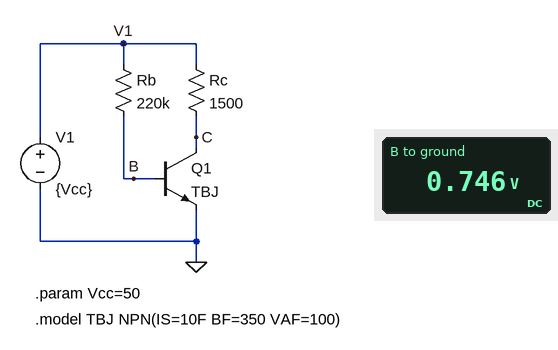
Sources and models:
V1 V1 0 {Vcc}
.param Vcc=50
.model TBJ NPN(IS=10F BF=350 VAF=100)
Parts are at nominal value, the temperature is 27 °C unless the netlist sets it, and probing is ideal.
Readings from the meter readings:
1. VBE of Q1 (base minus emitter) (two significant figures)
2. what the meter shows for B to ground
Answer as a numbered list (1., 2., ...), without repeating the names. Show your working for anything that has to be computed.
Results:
1. 746 mV = 750 mV
2. 0.746 V
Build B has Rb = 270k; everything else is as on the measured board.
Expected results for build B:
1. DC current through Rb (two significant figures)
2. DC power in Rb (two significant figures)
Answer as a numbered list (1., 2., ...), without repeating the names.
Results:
1. 180 µA
2. 9.0 mW
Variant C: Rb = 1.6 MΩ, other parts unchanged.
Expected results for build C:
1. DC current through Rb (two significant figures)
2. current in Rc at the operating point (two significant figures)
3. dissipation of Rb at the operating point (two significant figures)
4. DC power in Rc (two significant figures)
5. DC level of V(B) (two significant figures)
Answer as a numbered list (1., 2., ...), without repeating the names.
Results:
1. 31 µA
2. 14 mA
3. 1.5 mW
4. 290 mW
5. 720 mV
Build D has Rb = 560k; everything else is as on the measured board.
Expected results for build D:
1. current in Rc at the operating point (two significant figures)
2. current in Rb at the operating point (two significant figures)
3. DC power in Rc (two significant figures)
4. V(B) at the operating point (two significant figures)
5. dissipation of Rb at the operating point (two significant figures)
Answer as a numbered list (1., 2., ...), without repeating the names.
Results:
1. 31 mA
2. 88 µA
3. 1.5 W
4. 740 mV
5. 4.3 mW
